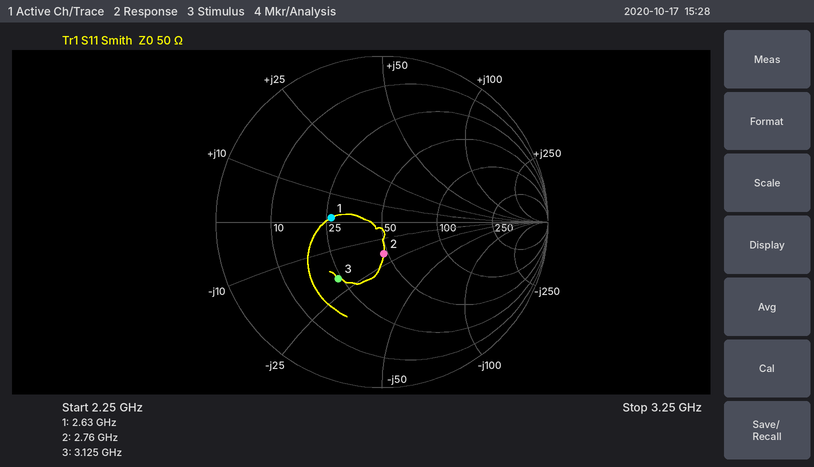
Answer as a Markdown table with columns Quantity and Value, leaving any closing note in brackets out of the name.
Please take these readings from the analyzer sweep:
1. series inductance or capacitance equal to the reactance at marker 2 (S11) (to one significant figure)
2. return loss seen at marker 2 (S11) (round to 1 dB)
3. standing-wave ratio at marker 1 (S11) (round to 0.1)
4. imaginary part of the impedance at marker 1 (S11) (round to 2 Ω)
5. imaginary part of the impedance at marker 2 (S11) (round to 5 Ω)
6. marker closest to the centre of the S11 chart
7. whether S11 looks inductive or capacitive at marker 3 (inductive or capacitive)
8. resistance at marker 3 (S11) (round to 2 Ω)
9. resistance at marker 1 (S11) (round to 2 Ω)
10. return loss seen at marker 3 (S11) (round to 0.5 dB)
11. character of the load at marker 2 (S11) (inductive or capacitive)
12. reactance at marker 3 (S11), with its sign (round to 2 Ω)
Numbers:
| Quantity | Value |
|---|---|
| series inductance or capacitance equal to the reactance at marker 2 (S11) | 3 pF |
| return loss seen at marker 2 (S11) | 14 dB |
| standing-wave ratio at marker 1 (S11) | 1.9 |
| imaginary part of the impedance at marker 1 (S11) | +2 Ω |
| imaginary part of the impedance at marker 2 (S11) | -20 Ω |
| marker closest to the centre of the S11 chart | marker 2 |
| whether S11 looks inductive or capacitive at marker 3 | capacitive |
| resistance at marker 3 (S11) | 24 Ω |
| resistance at marker 1 (S11) | 26 Ω |
| return loss seen at marker 3 (S11) | 7.5 dB |
| character of the load at marker 2 (S11) | capacitive |
| reactance at marker 3 (S11), with its sign | -20 Ω |
